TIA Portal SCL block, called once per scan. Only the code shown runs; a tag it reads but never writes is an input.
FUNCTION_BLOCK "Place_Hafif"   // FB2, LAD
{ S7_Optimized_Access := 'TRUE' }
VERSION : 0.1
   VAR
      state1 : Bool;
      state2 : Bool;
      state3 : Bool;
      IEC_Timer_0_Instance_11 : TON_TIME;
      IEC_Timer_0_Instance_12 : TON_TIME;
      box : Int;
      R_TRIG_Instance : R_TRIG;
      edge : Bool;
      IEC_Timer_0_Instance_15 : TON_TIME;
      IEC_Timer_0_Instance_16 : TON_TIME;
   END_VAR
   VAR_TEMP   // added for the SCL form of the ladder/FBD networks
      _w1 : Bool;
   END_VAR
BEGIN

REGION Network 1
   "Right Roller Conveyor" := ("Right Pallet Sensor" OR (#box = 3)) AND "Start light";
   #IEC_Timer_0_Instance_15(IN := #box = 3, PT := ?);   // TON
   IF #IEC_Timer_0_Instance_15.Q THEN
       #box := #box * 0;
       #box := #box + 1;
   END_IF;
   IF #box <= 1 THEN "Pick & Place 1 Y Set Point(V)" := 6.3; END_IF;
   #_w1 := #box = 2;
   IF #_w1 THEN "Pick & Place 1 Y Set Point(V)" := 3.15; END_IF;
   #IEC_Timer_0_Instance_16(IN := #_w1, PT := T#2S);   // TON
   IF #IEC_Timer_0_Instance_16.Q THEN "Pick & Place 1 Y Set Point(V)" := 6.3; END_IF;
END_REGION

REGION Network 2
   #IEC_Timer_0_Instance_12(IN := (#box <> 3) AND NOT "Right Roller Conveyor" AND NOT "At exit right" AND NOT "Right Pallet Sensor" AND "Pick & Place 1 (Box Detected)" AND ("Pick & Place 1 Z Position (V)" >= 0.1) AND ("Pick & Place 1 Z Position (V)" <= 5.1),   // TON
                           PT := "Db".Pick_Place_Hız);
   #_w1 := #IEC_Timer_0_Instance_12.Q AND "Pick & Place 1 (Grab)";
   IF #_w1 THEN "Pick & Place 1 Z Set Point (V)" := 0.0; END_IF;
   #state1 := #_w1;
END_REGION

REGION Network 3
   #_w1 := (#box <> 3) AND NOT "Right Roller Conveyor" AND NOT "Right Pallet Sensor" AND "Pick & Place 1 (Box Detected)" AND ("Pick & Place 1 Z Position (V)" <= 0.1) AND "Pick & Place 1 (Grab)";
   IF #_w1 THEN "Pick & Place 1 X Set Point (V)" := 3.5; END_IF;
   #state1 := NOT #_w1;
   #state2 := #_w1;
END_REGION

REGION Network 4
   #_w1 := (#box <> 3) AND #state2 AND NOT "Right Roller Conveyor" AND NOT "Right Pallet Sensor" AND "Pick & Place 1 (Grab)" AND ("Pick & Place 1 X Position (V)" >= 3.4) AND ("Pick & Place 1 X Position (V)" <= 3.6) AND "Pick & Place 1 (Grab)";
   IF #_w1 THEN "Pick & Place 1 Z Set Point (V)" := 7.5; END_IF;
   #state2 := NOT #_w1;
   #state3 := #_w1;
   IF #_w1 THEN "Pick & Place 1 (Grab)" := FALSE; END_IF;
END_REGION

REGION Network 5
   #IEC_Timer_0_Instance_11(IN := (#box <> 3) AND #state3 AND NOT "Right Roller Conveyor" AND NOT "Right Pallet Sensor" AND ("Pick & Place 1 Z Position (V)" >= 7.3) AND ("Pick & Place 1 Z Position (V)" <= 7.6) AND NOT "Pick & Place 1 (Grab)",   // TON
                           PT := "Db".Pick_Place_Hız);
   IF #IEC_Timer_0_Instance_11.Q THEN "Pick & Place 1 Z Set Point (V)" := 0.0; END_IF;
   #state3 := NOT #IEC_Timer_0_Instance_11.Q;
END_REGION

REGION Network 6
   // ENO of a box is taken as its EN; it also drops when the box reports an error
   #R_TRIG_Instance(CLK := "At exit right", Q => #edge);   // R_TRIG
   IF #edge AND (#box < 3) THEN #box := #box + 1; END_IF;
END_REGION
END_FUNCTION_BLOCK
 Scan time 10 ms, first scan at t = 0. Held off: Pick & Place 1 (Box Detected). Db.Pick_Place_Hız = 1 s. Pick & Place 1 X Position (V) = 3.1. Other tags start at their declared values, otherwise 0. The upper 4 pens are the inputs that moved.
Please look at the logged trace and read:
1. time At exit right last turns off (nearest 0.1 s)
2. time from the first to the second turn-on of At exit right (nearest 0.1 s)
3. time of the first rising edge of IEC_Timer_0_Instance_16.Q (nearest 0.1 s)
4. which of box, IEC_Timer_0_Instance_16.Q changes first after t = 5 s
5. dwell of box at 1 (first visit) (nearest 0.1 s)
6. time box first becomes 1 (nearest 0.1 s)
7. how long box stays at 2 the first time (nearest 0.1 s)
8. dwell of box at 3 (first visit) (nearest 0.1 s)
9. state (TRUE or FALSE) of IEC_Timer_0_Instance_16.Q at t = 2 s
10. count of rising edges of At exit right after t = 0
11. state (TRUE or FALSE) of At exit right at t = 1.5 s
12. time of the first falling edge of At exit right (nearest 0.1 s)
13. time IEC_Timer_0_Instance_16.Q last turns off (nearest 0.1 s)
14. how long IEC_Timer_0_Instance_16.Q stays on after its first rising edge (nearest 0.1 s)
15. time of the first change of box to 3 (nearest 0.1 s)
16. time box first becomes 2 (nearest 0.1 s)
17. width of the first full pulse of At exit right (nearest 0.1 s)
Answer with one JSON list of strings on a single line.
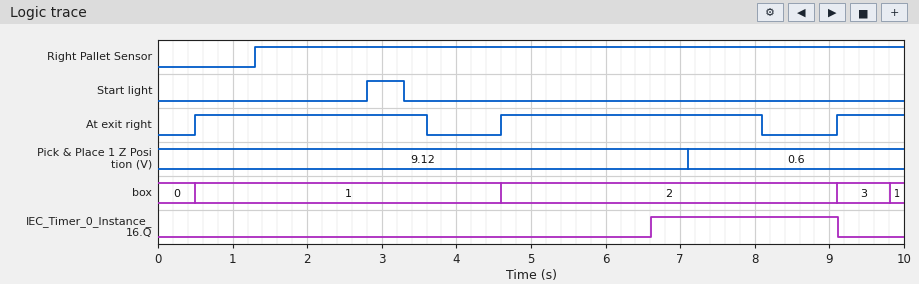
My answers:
["8.1 s", "4.1 s", "6.6 s", "IEC_Timer_0_Instance_16.Q", "4.1 s", "0.5 s", "4.5 s", "0.7 s", "FALSE", "3", "TRUE", "3.6 s", "9.1 s", "2.5 s", "9.1 s", "4.6 s", "3.1 s"]
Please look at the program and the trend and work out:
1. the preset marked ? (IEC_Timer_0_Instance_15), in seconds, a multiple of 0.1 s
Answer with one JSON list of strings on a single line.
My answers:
["0.7 s"]
